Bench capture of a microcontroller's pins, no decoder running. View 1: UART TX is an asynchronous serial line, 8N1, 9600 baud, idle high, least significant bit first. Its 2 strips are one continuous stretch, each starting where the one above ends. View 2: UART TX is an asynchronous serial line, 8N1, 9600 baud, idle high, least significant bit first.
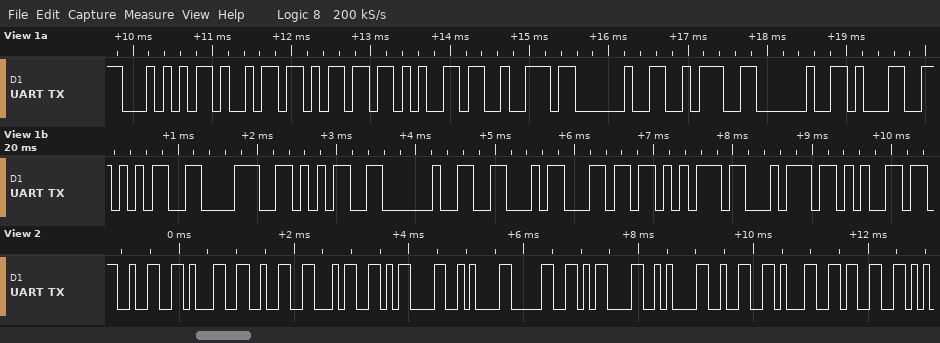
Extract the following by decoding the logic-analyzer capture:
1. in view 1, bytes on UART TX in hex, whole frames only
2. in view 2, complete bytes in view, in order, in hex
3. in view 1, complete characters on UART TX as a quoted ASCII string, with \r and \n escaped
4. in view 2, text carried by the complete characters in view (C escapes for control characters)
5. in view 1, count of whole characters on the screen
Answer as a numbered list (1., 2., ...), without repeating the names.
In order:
1. 54 69 6D 65 72 20 3A 20 31 35 38 35 20 46 6C 75 74 65
2. 32 31 32 34 0D 0A 30 0D 0A 32 31 33
3. "Timer : 1585 Flute"
4. "2124\r\n0\r\n213"
5. 18
